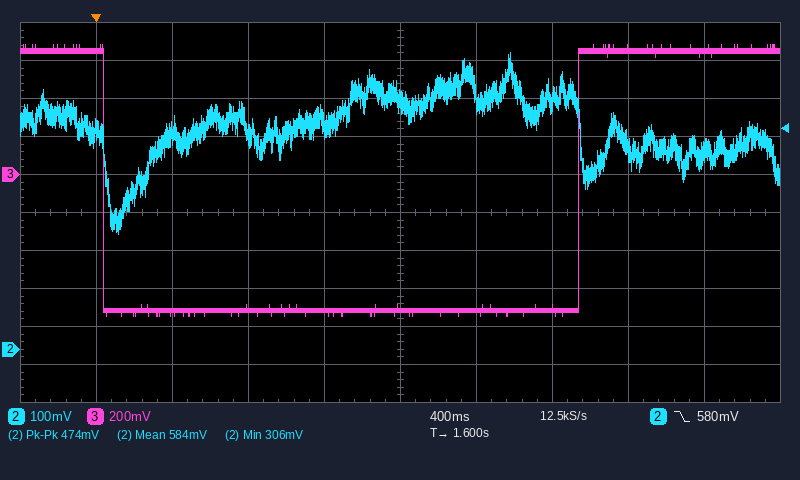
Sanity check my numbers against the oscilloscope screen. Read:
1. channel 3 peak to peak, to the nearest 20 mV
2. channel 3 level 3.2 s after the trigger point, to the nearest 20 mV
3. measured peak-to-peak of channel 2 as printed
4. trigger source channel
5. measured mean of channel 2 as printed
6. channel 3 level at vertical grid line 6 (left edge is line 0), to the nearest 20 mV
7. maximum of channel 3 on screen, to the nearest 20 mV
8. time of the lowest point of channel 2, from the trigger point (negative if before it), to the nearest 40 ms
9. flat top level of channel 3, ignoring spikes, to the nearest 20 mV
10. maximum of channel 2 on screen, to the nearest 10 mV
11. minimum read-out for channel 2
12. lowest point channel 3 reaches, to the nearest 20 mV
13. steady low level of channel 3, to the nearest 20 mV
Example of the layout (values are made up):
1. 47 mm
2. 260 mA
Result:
1. 1.42 V
2. 660 mV
3. 474 mV
4. channel 2
5. 584 mV
6. -720 mV
7. 680 mV
8. +120 ms
9. 660 mV
10. 780 mV
11. 306 mV
12. -740 mV
13. -720 mV
